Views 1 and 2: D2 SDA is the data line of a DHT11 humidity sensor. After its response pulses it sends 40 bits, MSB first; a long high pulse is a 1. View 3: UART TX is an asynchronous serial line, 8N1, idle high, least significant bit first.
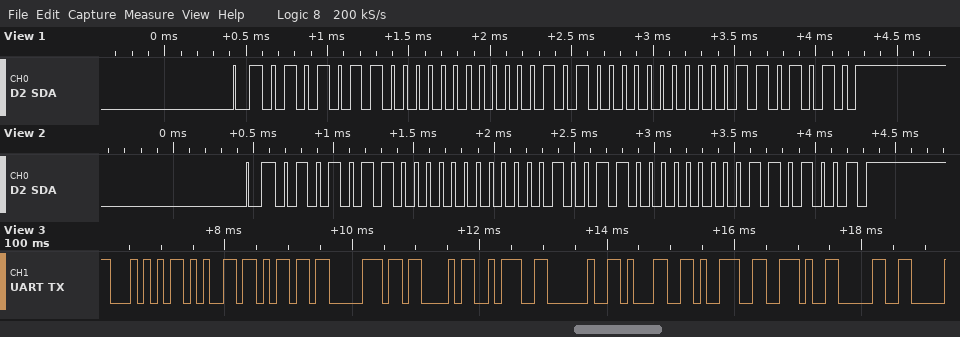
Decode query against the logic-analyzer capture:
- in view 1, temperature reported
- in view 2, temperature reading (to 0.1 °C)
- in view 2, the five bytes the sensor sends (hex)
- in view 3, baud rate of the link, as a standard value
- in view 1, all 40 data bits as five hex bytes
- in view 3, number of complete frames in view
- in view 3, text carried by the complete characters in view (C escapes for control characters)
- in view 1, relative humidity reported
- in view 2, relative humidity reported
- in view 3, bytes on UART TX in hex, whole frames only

20.0 °C
19.0 °C
56 00 13 00 69
9600 baud
56 00 14 00 6A
11
"TempC: 19.0"
86 %
86 %
54 65 6D 70 43 3A 20 31 39 2E 30
